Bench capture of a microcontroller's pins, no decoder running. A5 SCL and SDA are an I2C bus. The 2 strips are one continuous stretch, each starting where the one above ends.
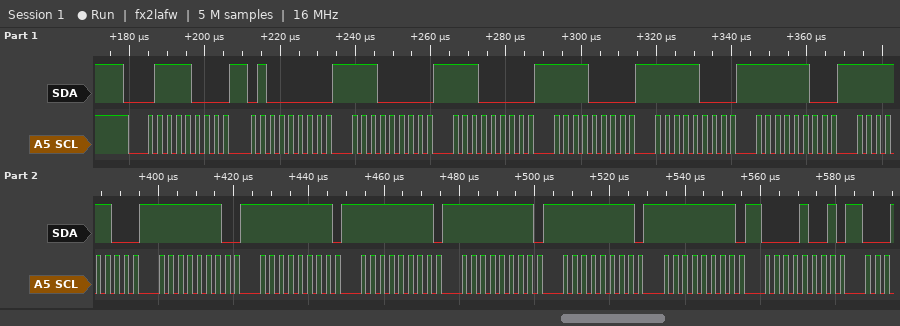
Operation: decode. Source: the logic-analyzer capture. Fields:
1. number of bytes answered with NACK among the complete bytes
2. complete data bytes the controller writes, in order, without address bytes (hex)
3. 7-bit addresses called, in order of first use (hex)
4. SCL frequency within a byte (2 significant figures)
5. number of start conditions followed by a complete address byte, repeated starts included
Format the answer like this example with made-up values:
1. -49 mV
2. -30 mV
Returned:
1. 0
2. 40 E0 E0 F0 F8 FC FC FE FF FF FF FF FF 09
3. 0x3C
4. 400 kHz
5. 1
